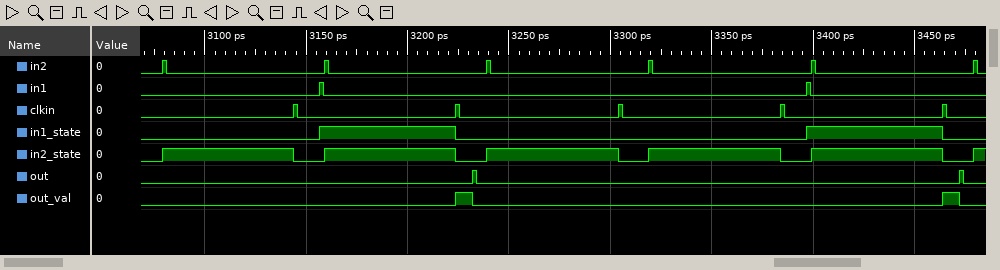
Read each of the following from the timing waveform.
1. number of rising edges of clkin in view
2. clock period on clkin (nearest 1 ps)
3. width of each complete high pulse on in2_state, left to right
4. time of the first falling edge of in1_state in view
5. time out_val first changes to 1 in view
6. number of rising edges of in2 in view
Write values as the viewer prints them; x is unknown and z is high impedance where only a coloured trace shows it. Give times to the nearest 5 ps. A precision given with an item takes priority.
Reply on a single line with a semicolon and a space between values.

5; 80 ps; 65 ps, 65 ps, 65 ps, 65 ps, 65 ps; 3225 ps; 3225 ps; 6
